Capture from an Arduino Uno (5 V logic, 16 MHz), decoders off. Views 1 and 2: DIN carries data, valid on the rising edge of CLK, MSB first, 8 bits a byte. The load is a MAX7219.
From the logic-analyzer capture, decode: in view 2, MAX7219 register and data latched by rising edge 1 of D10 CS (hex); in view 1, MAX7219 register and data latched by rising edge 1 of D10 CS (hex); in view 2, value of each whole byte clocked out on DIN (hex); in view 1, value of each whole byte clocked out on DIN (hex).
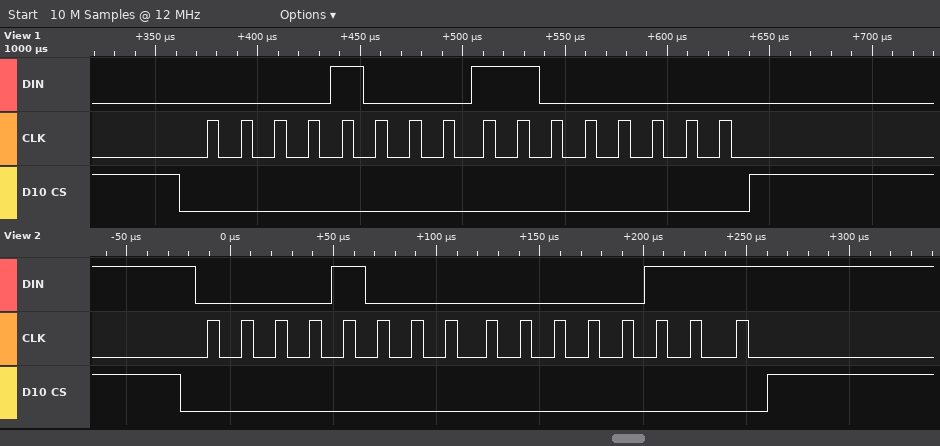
register 0x8, data 0x07
register 0x8, data 0xC0
0x08 0x07
0x08 0xC0
